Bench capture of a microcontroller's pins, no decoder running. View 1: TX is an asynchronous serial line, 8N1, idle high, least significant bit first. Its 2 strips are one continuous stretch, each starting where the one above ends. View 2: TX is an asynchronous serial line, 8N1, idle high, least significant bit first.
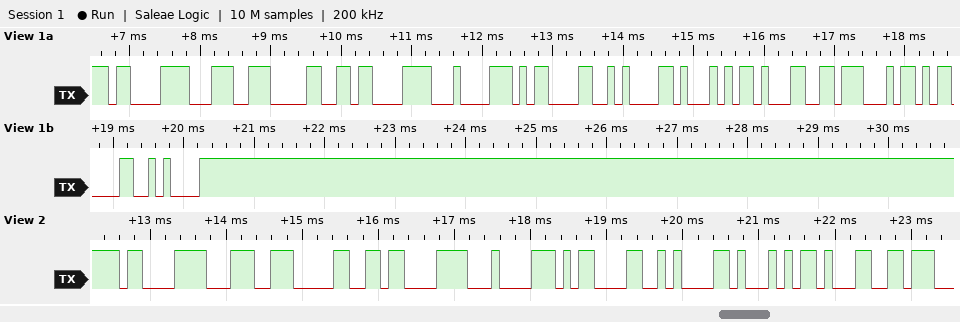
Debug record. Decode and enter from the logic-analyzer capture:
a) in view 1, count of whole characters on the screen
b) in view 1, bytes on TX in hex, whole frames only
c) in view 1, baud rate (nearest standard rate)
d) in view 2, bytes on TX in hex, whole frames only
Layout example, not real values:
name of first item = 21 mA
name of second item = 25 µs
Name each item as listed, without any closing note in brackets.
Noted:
in view 1, count of whole characters on the screen = 12
in view 1, bytes on TX in hex, whole frames only = C3 9C 30 C3 84 0D 0A 51 31 47 0D 0A
in view 1, baud rate = 9600 baud
in view 2, bytes on TX in hex, whole frames only = C3 9C 30 C3 84 0D 0A 51 31
